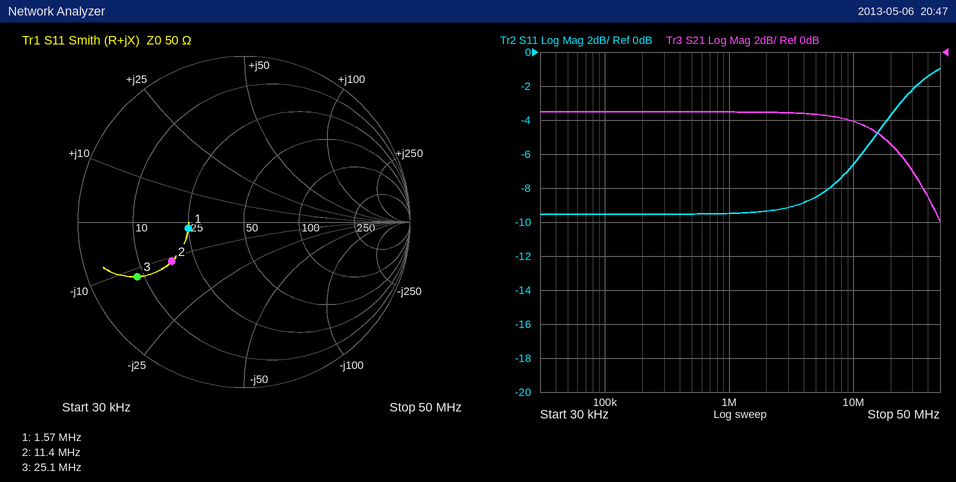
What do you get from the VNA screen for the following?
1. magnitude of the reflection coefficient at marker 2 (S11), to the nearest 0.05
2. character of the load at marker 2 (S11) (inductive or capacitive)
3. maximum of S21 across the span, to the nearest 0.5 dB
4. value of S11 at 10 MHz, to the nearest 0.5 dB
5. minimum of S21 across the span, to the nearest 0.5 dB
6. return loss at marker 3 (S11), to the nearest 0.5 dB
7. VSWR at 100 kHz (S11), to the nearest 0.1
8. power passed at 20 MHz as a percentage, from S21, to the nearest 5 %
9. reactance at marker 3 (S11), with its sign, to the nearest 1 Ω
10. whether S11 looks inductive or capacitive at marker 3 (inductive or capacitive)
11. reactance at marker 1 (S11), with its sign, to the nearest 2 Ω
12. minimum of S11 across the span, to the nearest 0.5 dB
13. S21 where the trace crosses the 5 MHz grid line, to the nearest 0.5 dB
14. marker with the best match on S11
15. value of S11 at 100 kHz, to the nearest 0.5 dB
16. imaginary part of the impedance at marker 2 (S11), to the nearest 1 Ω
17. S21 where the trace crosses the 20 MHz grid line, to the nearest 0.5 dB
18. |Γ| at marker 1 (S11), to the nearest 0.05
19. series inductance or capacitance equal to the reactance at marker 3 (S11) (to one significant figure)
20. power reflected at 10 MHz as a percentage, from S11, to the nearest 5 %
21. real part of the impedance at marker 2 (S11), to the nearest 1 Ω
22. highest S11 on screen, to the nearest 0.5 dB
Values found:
0.50
capacitive
-3.5 dB
-6.5 dB
-10.0 dB
3.0 dB
2.0
30 %
-12 Ω
capacitive
-2 Ω
-9.5 dB
-3.5 dB
marker 1
-9.5 dB
-11 Ω
-5.5 dB
0.35
500 pF
20 %
18 Ω
-1.0 dB
